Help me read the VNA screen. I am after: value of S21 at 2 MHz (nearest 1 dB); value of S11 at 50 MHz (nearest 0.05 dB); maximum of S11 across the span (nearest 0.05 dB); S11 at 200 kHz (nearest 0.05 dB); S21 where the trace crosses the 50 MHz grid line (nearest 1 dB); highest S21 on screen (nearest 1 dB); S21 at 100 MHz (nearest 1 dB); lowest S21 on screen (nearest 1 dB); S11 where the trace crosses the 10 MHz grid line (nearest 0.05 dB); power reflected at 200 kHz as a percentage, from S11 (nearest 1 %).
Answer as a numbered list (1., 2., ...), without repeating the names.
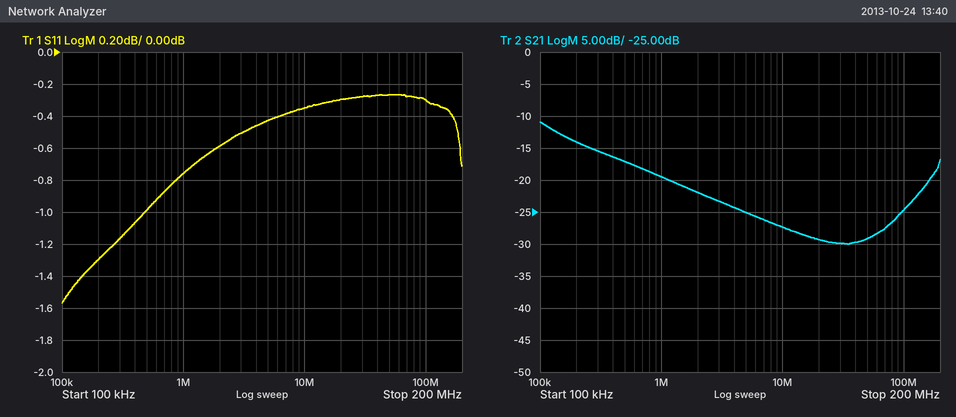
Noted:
1. -22 dB
2. -0.25 dB
3. -0.25 dB
4. -1.30 dB
5. -29 dB
6. -11 dB
7. -25 dB
8. -30 dB
9. -0.35 dB
10. 74 %
